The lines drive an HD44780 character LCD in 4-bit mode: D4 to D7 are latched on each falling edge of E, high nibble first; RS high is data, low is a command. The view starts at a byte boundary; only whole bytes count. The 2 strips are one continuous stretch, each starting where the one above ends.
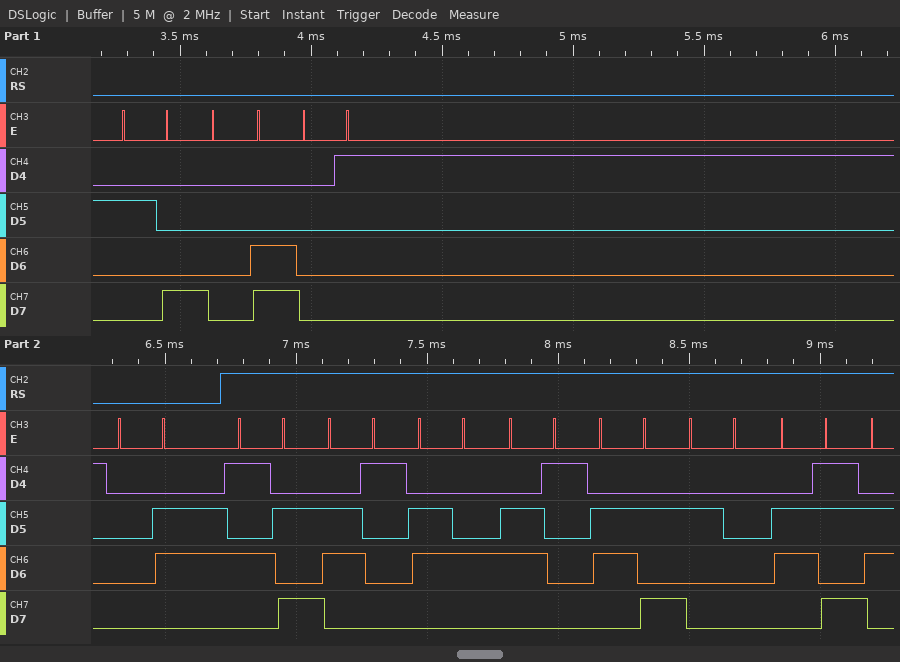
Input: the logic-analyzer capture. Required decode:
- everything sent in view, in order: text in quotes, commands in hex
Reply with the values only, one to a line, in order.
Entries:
0x28 0x0C 0x01 0x06 "Zadaj k"
